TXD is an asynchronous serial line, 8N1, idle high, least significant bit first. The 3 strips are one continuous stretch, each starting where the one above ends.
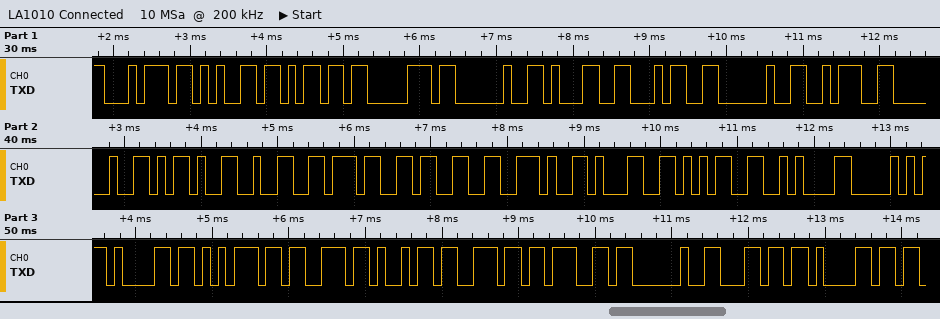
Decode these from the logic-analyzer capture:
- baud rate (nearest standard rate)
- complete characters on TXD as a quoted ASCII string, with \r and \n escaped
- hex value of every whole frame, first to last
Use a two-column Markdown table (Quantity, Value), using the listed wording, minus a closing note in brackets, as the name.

| Quantity | Value |
|---|---|
| baud rate | 9600 baud |
| complete characters on TXD as a quoted ASCII string, with \r and \n escaped | "temp 14 : -273.15\nPausing la" |
| hex value of every whole frame, first to last | 74 65 6D 70 20 31 34 20 3A 20 2D 32 37 33 2E 31 35 0A 50 61 75 73 69 6E 67 20 6C 61 |
